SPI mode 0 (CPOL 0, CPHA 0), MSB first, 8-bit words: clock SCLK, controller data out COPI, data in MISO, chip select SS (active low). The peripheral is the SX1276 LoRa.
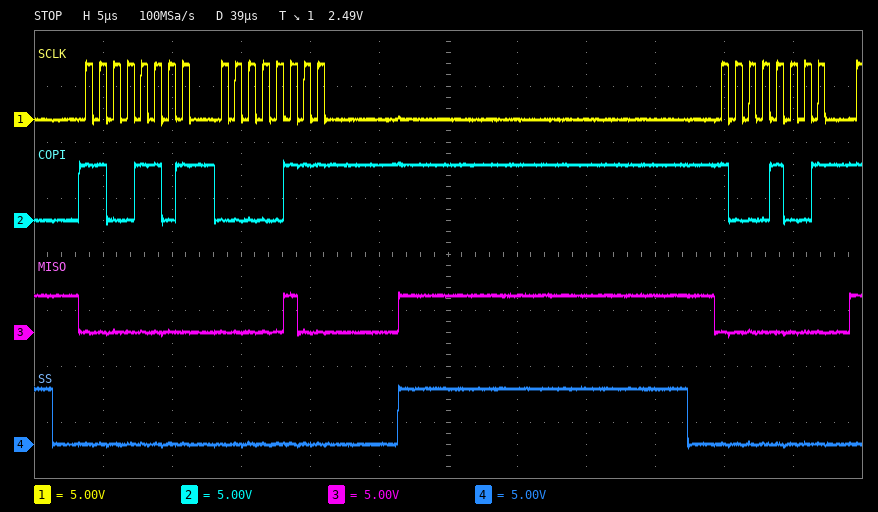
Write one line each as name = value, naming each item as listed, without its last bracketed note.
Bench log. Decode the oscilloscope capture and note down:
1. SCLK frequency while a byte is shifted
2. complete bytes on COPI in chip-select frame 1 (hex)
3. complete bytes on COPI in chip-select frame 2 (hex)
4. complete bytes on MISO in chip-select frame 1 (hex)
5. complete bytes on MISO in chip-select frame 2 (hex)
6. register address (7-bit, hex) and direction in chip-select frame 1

SCLK frequency while a byte is shifted = 1 MHz
complete bytes on COPI in chip-select frame 1 = CD 07
complete bytes on COPI in chip-select frame 2 = 89
complete bytes on MISO in chip-select frame 1 = 00 04
complete bytes on MISO in chip-select frame 2 = 00
register address (7-bit, hex) and direction in chip-select frame 1 = 0x4D write
